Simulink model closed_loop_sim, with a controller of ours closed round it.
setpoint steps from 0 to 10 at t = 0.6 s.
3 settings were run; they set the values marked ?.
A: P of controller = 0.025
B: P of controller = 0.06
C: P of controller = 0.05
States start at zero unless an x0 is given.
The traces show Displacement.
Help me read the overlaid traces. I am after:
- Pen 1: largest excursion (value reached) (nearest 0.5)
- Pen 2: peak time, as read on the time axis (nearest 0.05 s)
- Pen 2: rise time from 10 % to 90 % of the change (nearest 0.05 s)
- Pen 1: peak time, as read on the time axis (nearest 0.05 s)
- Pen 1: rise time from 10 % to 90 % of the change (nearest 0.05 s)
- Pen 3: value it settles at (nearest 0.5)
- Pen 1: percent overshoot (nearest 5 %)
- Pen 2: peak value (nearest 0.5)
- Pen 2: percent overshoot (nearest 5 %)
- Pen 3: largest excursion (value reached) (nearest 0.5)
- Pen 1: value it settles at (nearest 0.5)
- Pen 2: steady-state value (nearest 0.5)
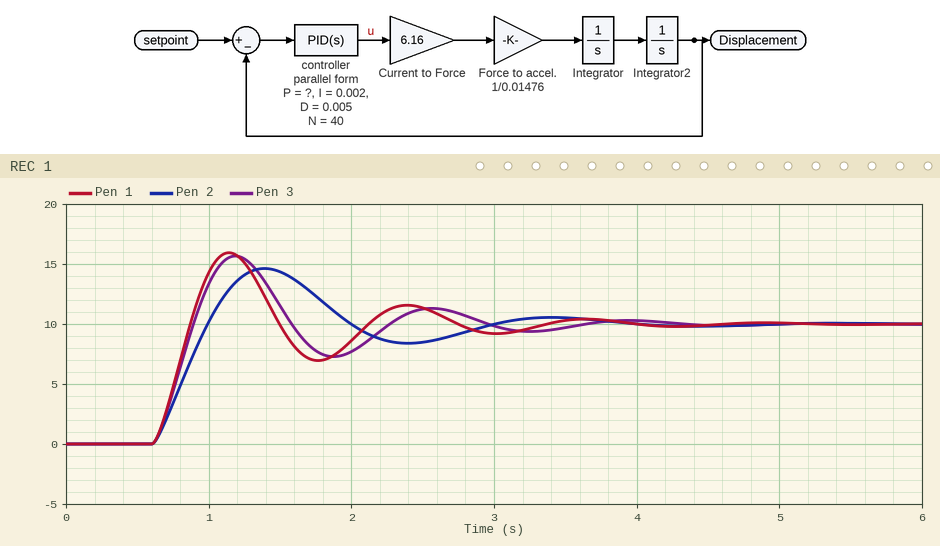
16.0
1.40 s
0.30 s
1.15 s
0.20 s
10.0
60 %
14.5
45 %
15.5
10.0
10.0
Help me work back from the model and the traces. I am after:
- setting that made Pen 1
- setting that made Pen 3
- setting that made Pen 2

B
C
A
